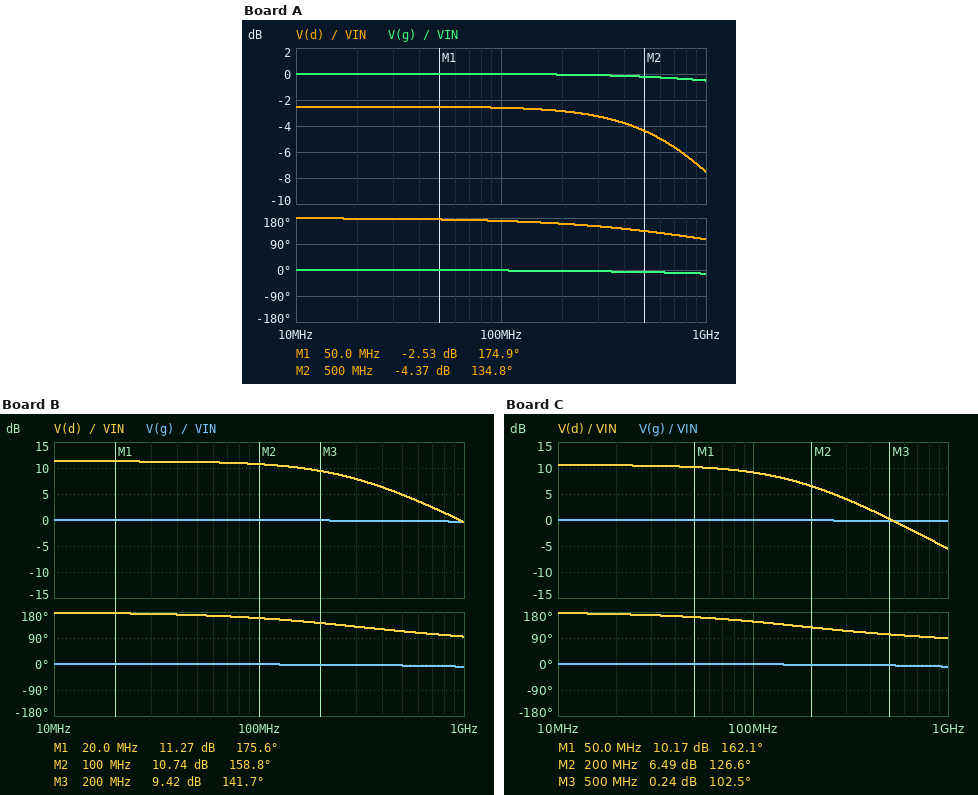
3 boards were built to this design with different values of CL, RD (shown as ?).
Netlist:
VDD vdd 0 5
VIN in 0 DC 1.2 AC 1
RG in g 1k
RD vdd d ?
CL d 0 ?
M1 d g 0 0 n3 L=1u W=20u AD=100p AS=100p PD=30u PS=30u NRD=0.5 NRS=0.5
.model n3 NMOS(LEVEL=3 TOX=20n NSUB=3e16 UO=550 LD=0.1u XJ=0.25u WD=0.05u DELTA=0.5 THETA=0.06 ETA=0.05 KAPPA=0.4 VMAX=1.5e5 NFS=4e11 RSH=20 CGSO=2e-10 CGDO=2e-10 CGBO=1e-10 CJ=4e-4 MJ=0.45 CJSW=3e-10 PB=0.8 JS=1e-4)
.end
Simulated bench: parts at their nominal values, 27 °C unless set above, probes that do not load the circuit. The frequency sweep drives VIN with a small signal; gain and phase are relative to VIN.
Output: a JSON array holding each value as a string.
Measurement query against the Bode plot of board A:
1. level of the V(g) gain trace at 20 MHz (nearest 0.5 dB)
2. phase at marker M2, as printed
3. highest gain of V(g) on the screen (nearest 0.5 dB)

["0 dB", "134.8 deg", "0 dB"]
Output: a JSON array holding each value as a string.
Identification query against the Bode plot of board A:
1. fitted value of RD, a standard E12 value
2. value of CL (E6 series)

["8.2 kΩ", "150 fF"]
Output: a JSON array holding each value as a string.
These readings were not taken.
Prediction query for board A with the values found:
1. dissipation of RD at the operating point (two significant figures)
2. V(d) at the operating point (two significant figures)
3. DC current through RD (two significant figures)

["2.6 mW", "400 mV", "560 µA"]
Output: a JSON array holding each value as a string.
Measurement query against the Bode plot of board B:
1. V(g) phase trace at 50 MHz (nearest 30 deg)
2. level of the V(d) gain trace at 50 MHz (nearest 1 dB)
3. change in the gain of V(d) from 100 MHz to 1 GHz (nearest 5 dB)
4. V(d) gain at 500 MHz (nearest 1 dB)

["0 deg", "11 dB", "-10 dB", "5 dB"]
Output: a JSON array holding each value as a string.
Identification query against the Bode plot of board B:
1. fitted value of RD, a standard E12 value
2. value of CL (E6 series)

["4.7 kΩ", "150 fF"]
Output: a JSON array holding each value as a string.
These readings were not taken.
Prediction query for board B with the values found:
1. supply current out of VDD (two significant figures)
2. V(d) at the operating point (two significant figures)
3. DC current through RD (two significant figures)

["780 µA", "1.3 V", "780 µA"]
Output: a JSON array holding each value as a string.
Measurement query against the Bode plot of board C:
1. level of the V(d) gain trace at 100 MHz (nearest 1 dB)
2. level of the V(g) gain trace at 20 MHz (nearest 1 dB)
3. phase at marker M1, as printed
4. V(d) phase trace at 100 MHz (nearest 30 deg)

["9 dB", "0 dB", "162.1 deg", "150 deg"]
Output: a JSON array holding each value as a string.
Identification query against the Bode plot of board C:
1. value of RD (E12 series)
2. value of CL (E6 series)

["3.9 kΩ", "330 fF"]
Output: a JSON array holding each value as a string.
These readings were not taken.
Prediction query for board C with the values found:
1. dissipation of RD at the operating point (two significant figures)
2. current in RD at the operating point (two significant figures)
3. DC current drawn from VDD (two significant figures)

["2.7 mW", "830 µA", "830 µA"]
